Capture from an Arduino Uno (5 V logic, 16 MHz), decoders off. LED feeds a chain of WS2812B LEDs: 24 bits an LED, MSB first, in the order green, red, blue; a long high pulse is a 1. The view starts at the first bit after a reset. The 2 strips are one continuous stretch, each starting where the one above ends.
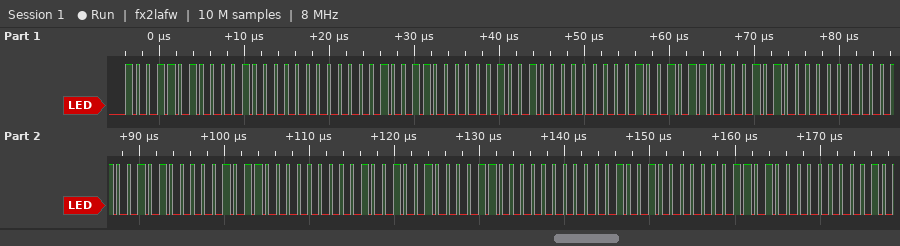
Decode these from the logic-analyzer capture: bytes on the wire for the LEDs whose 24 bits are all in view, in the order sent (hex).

9A 10 00 98 12 00 96 14 00 94 16 00 92 18 00 90 1A 00
